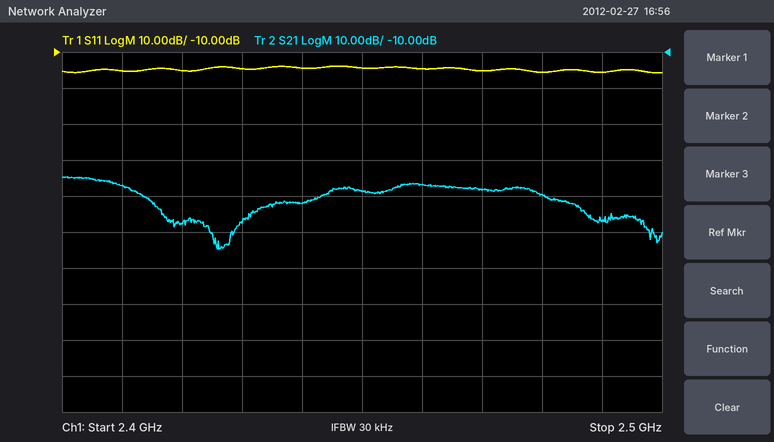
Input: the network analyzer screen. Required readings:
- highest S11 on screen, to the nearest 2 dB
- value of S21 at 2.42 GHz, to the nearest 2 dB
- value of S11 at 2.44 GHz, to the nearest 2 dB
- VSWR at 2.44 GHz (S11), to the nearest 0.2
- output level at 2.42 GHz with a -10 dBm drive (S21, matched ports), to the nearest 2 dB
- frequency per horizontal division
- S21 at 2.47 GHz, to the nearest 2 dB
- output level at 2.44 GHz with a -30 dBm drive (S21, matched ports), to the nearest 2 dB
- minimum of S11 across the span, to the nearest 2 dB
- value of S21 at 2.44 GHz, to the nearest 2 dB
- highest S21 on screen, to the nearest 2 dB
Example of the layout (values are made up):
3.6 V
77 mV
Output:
-14 dB
-58 dB
-14 dB
1.4
-68 dBm
10 MHz
-48 dB
-82 dBm
-16 dB
-52 dB
-44 dB
